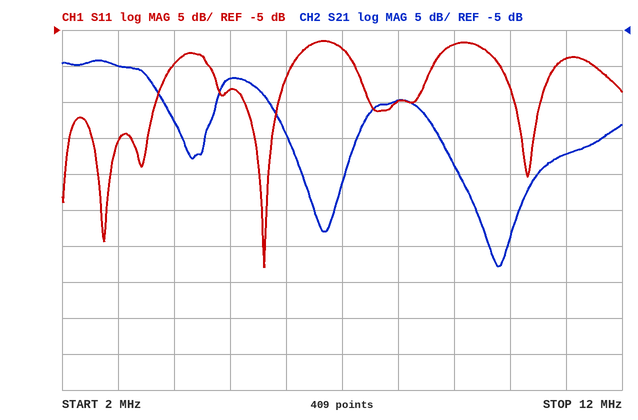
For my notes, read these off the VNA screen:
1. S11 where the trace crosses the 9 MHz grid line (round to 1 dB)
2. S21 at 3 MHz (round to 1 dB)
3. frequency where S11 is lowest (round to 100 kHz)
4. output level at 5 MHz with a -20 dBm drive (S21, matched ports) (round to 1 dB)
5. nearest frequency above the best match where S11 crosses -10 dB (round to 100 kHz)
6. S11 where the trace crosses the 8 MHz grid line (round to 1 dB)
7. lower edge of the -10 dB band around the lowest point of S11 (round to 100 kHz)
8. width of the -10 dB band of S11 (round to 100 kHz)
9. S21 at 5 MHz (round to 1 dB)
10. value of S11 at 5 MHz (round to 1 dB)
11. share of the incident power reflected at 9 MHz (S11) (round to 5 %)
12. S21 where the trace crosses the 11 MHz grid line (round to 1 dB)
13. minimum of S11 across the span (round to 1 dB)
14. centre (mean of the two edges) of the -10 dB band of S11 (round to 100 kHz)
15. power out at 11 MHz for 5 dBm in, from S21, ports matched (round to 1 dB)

-7 dB
-10 dB
5.6 MHz
-32 dBm
6.1 MHz
-15 dB
4.6 MHz
1.5 MHz
-12 dB
-13 dB
20 %
-22 dB
-38 dB
5.4 MHz
-17 dBm
